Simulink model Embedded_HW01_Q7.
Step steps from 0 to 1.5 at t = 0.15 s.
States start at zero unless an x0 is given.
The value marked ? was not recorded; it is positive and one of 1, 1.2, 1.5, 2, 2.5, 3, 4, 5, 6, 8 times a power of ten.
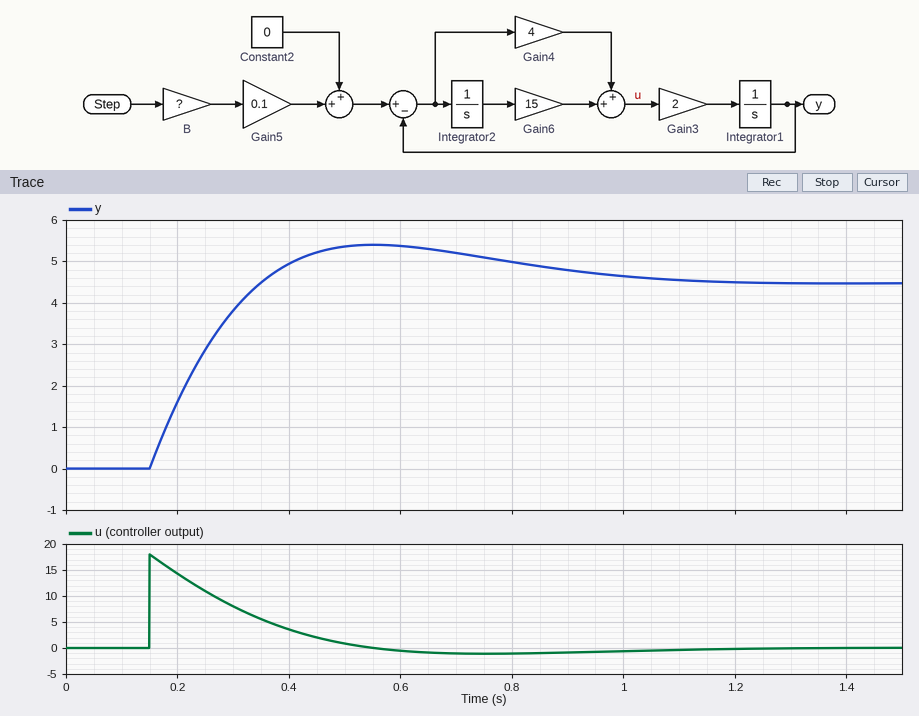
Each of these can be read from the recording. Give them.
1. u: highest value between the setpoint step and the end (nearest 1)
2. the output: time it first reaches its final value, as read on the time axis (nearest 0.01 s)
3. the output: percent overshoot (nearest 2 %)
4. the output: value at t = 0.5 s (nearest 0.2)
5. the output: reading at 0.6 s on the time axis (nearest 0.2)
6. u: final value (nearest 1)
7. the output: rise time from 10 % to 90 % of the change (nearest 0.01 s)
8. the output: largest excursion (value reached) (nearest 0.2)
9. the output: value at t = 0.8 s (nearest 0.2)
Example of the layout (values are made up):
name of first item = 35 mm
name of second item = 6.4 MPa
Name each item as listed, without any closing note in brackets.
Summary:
u: highest value between the setpoint step and the end = 18
the output: time it first reaches its final value, as read on the time axis = 0.35 s
the output: percent overshoot = 20 %
the output: value at t = 0.5 s = 5.4
the output: reading at 0.6 s on the time axis = 5.4
u: final value = 0
the output: rise time from 10 % to 90 % of the change = 0.15 s
the output: largest excursion (value reached) = 5.4
the output: value at t = 0.8 s = 5.0
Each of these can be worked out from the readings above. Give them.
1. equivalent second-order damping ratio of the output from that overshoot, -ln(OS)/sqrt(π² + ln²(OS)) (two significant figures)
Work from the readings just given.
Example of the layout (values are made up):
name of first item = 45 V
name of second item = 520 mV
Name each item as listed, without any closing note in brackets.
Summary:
equivalent second-order damping ratio of the output from that overshoot, -ln(OS)/sqrt(π² + ln²(OS)) = 0.46
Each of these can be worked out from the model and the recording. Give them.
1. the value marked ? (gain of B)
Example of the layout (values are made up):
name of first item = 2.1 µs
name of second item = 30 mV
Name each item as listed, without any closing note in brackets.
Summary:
the value marked ? = 30
